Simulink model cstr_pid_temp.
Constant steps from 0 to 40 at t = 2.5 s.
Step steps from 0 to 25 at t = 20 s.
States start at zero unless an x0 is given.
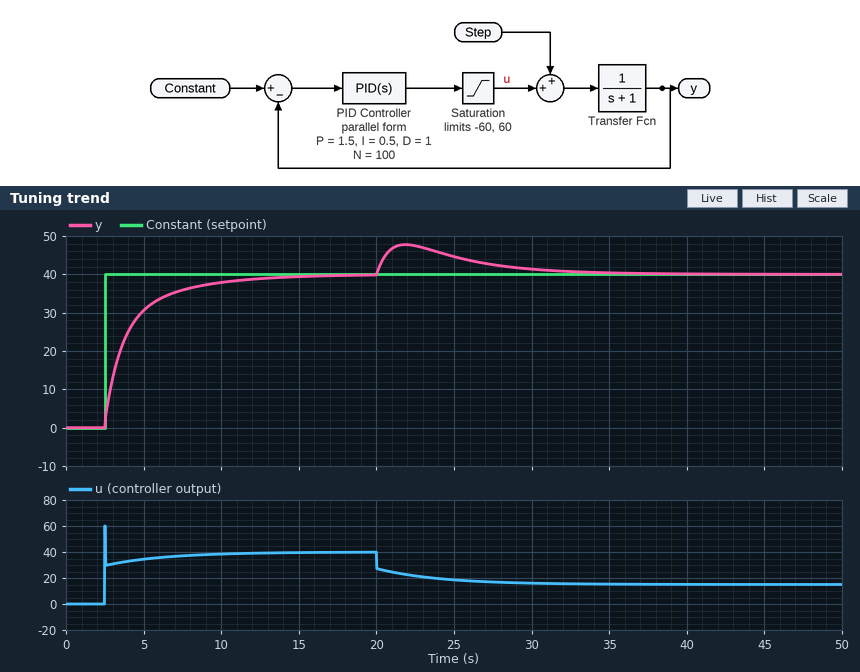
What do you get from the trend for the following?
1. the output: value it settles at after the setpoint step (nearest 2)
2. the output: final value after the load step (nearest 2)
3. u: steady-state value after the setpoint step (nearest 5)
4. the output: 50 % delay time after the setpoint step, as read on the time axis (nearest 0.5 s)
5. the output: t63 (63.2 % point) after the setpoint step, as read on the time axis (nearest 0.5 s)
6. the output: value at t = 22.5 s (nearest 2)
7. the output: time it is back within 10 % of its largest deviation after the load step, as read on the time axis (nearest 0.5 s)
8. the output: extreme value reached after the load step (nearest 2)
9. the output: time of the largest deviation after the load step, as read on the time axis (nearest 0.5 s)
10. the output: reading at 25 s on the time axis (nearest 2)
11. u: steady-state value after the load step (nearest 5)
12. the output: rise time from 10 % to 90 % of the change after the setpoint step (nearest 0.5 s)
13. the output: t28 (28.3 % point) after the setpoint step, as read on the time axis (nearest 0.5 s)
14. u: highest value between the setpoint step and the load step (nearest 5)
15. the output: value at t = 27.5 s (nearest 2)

40
40
40
3.5 s
4.0 s
48
32.0 s
48
22.0 s
44
15
5.0 s
3.0 s
60
42
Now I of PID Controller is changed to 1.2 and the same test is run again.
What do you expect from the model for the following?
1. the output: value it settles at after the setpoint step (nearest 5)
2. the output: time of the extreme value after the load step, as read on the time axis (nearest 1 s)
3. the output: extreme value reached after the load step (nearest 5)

40
21 s
45
